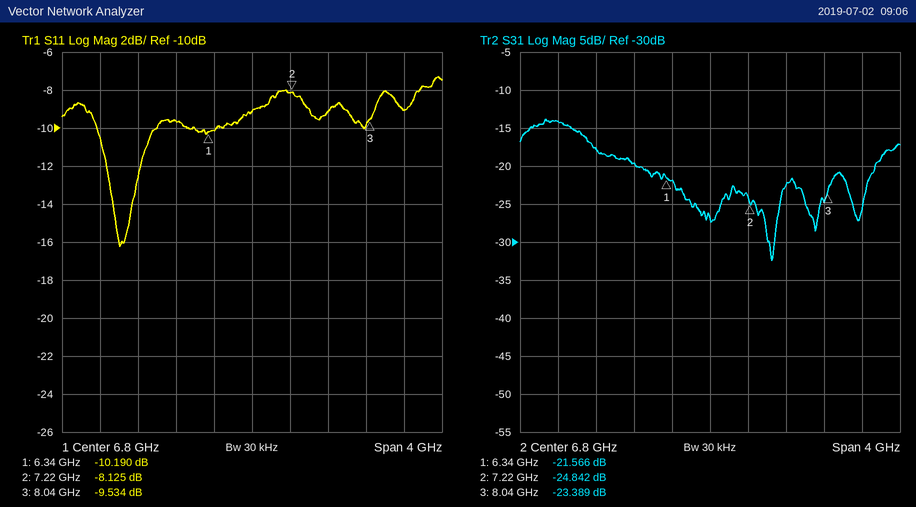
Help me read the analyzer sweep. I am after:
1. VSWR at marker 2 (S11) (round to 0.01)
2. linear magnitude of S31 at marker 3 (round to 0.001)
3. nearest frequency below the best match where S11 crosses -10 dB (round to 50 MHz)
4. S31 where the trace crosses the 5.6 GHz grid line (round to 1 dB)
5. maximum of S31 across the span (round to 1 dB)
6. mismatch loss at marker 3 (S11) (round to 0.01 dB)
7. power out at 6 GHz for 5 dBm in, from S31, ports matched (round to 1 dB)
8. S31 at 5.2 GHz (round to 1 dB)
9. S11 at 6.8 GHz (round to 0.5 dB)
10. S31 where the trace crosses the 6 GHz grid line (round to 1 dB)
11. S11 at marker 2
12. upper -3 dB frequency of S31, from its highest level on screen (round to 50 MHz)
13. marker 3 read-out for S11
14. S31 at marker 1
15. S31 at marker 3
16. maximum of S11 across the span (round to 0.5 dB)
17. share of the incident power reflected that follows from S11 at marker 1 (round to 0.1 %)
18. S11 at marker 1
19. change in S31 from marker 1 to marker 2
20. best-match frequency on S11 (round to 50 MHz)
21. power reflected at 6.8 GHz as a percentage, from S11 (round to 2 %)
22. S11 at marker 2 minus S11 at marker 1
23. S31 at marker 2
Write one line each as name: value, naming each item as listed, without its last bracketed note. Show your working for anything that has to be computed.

VSWR at marker 2 (S11): (1 + 0.3924)/(1 − 0.3924) ≈ 2.29
linear magnitude of S31 at marker 3: 10^(-23.389/20) ≈ 0.068
nearest frequency below the best match where S11 crosses -10 dB: 5.15 GHz
S31 where the trace crosses the 5.6 GHz grid line: -18 dB
maximum of S31 across the span: -14 dB
mismatch loss at marker 3 (S11): −10 log10(1 − 10^(-9.534/10)) ≈ 0.51 dB
power out at 6 GHz for 5 dBm in, from S31, ports matched: 5 dBm + (-20 dB) = -15 dBm
S31 at 5.2 GHz: -14 dB
S11 at 6.8 GHz: -9.0 dB
S31 where the trace crosses the 6 GHz grid line: -20 dB
S11 at marker 2: -8.125 dB
upper -3 dB frequency of S31, from its highest level on screen: 5.55 GHz
marker 3 read-out for S11: -9.534 dB
S31 at marker 1: -21.566 dB
S31 at marker 3: -23.389 dB
maximum of S11 across the span: -7.5 dB
share of the incident power reflected that follows from S11 at marker 1: 10^(-10.19/10) ≈ 9.6 %
S11 at marker 1: -10.190 dB
change in S31 from marker 1 to marker 2: -24.842 − (-21.566) = -3.276 dB
best-match frequency on S11: 5.40 GHz
power reflected at 6.8 GHz as a percentage, from S11: 10^(-9/10) ≈ 12.6 %, so 12 % to the nearest 2 %
S11 at marker 2 minus S11 at marker 1: -8.125 − (-10.19) = 2.065 dB
S31 at marker 2: -24.842 dB
